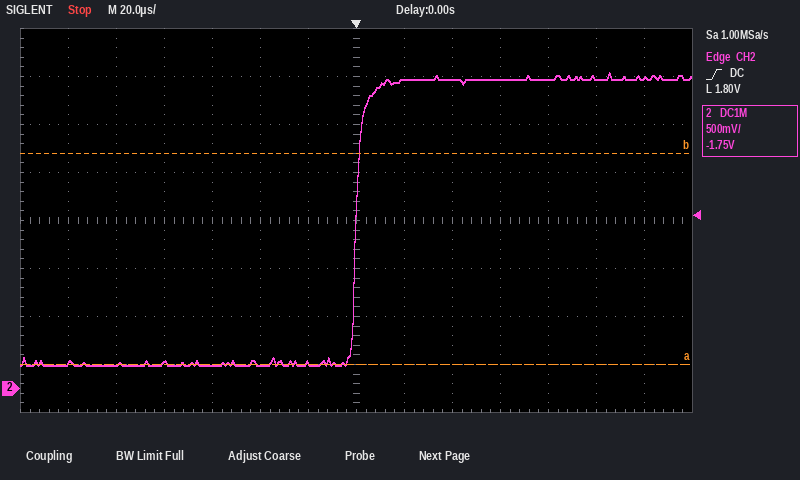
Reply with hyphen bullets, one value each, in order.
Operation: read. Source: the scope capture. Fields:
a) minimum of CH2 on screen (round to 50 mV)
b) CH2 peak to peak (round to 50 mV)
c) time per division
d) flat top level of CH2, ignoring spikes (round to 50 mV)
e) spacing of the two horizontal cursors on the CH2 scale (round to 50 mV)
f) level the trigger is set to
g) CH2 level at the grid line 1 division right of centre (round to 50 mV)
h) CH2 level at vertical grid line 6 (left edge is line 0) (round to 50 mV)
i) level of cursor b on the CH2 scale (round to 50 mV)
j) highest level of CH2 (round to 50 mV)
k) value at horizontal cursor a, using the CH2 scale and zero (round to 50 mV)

- 250 mV
- 3.05 V
- 20 µs
- 3.20 V
- 2.20 V
- 1.80 V
- 3.20 V
- 250 mV
- 2.45 V
- 3.30 V
- 250 mV
